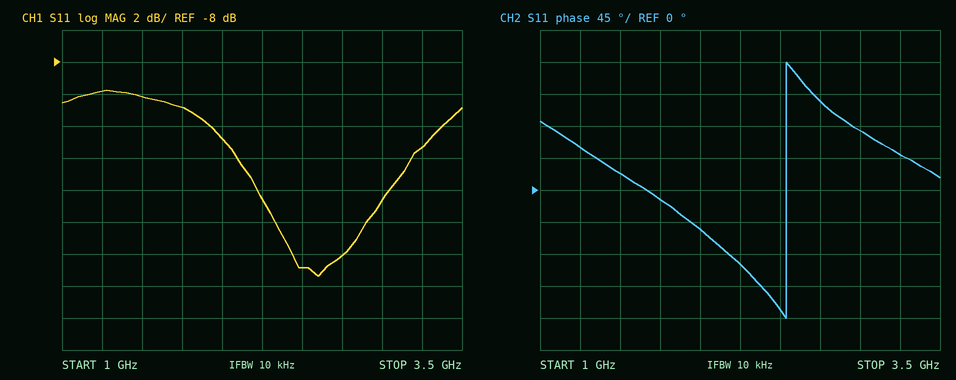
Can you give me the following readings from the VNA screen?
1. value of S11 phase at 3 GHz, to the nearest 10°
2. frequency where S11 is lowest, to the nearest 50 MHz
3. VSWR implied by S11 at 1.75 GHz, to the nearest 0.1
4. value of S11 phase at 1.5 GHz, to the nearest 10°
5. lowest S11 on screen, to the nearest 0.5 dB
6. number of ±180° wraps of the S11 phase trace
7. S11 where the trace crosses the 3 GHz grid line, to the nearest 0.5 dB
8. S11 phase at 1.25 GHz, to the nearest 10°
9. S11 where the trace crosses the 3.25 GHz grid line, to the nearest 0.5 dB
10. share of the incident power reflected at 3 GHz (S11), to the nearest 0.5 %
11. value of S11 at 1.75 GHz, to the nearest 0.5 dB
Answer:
80°
2.60 GHz
1.8
20°
-21.5 dB
1
-16.5 dB
60°
-13.5 dB
2.0 %
-11.0 dB
